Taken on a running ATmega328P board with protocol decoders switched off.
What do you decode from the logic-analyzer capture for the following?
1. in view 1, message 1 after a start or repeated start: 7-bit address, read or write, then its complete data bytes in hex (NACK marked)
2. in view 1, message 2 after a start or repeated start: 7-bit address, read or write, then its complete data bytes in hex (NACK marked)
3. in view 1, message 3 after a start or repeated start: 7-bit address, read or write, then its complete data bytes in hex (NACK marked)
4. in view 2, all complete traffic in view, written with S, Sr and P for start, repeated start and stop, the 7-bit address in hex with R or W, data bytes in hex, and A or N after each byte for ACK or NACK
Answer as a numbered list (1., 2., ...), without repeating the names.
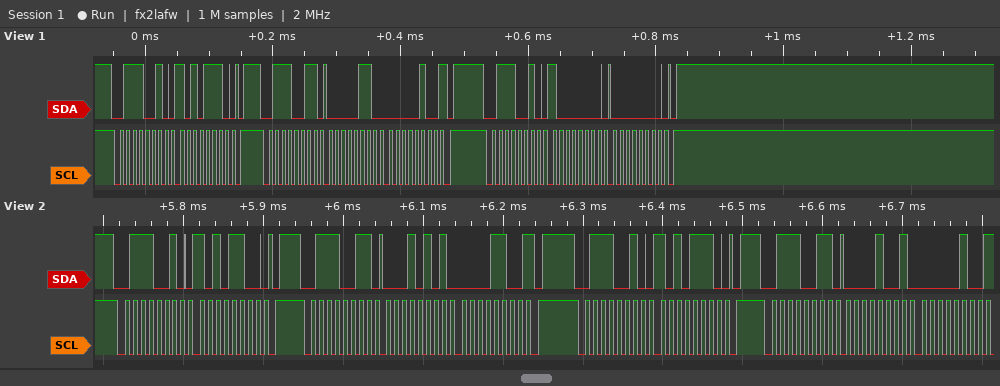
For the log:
1. 0x39 write: AE
2. 0x39 read: 06 04 NACK
3. 0x39 write: 80 00
4. S 39W A AC A P S 39R A 15 A 0C N P S 39W A AE A P S 39R A 09 A 04 N
